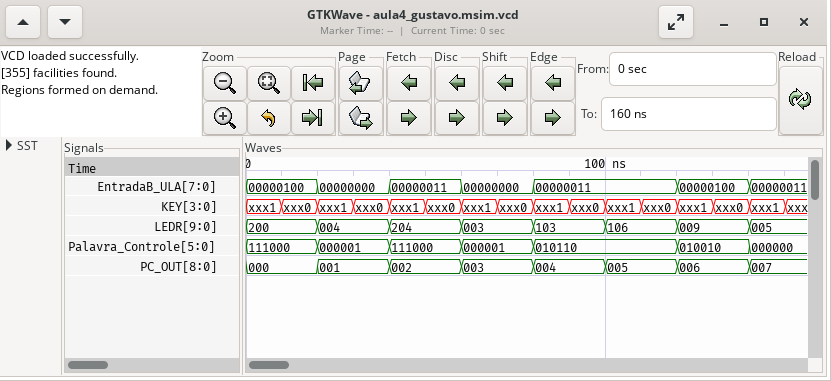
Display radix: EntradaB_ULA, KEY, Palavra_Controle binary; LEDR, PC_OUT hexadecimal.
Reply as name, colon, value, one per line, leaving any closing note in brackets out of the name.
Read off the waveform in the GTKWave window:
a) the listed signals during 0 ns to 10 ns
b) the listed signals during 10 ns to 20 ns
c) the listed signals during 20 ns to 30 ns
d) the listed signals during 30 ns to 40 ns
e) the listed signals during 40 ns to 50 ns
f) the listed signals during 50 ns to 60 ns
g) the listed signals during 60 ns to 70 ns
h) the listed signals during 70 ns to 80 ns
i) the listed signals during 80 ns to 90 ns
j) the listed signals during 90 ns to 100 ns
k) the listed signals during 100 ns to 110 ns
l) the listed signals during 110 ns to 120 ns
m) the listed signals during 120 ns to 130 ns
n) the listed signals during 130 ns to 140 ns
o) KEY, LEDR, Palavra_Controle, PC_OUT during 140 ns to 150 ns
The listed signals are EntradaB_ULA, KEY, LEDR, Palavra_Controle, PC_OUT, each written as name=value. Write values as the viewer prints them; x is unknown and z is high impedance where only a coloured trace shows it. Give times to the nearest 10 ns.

the listed signals during 0 ns to 10 ns: EntradaB_ULA=00000100, KEY=xxx1, LEDR=200, Palavra_Controle=111000, PC_OUT=000
the listed signals during 10 ns to 20 ns: EntradaB_ULA=00000100, KEY=xxx0, LEDR=200, Palavra_Controle=111000, PC_OUT=000
the listed signals during 20 ns to 30 ns: EntradaB_ULA=00000000, KEY=xxx1, LEDR=004, Palavra_Controle=000001, PC_OUT=001
the listed signals during 30 ns to 40 ns: EntradaB_ULA=00000000, KEY=xxx0, LEDR=004, Palavra_Controle=000001, PC_OUT=001
the listed signals during 40 ns to 50 ns: EntradaB_ULA=00000011, KEY=xxx1, LEDR=204, Palavra_Controle=111000, PC_OUT=002
the listed signals during 50 ns to 60 ns: EntradaB_ULA=00000011, KEY=xxx0, LEDR=204, Palavra_Controle=111000, PC_OUT=002
the listed signals during 60 ns to 70 ns: EntradaB_ULA=00000000, KEY=xxx1, LEDR=003, Palavra_Controle=000001, PC_OUT=003
the listed signals during 70 ns to 80 ns: EntradaB_ULA=00000000, KEY=xxx0, LEDR=003, Palavra_Controle=000001, PC_OUT=003
the listed signals during 80 ns to 90 ns: EntradaB_ULA=00000011, KEY=xxx1, LEDR=103, Palavra_Controle=010110, PC_OUT=004
the listed signals during 90 ns to 100 ns: EntradaB_ULA=00000011, KEY=xxx0, LEDR=103, Palavra_Controle=010110, PC_OUT=004
the listed signals during 100 ns to 110 ns: EntradaB_ULA=00000011, KEY=xxx1, LEDR=106, Palavra_Controle=010110, PC_OUT=005
the listed signals during 110 ns to 120 ns: EntradaB_ULA=00000011, KEY=xxx0, LEDR=106, Palavra_Controle=010110, PC_OUT=005
the listed signals during 120 ns to 130 ns: EntradaB_ULA=00000100, KEY=xxx1, LEDR=009, Palavra_Controle=010010, PC_OUT=006
the listed signals during 130 ns to 140 ns: EntradaB_ULA=00000100, KEY=xxx0, LEDR=009, Palavra_Controle=010010, PC_OUT=006
KEY, LEDR, Palavra_Controle, PC_OUT during 140 ns to 150 ns: KEY=xxx1, LEDR=005, Palavra_Controle=000000, PC_OUT=007
